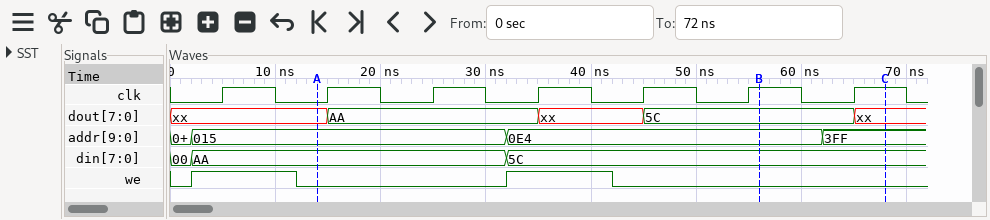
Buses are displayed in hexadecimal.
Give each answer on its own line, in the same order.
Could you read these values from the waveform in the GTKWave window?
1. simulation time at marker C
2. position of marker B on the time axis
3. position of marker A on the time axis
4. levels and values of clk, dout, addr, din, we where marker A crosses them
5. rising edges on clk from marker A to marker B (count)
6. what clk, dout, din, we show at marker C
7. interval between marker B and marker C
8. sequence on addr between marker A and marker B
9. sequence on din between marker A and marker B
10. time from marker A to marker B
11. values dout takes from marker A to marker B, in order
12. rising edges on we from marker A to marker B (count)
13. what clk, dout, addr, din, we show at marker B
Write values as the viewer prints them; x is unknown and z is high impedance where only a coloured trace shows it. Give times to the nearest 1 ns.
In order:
68 ns
56 ns
14 ns
clk=0, dout=xx, addr=015, din=AA, we=0
5
clk=1, dout=xx, din=5C, we=0
12 ns
015, 0E4
AA, 5C
42 ns
xx, AA, xx, 5C
1
clk=1, dout=5C, addr=0E4, din=5C, we=0
